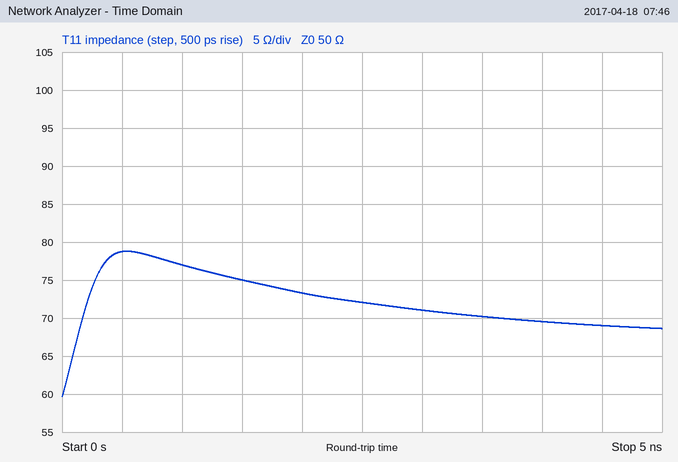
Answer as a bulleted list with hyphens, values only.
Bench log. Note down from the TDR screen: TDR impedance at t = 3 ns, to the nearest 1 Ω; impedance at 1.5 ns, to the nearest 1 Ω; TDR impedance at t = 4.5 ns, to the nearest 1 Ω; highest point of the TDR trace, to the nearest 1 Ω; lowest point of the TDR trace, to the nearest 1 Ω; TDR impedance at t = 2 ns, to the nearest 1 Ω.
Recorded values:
- 71 Ω
- 75 Ω
- 69 Ω
- 79 Ω
- 60 Ω
- 73 Ω
